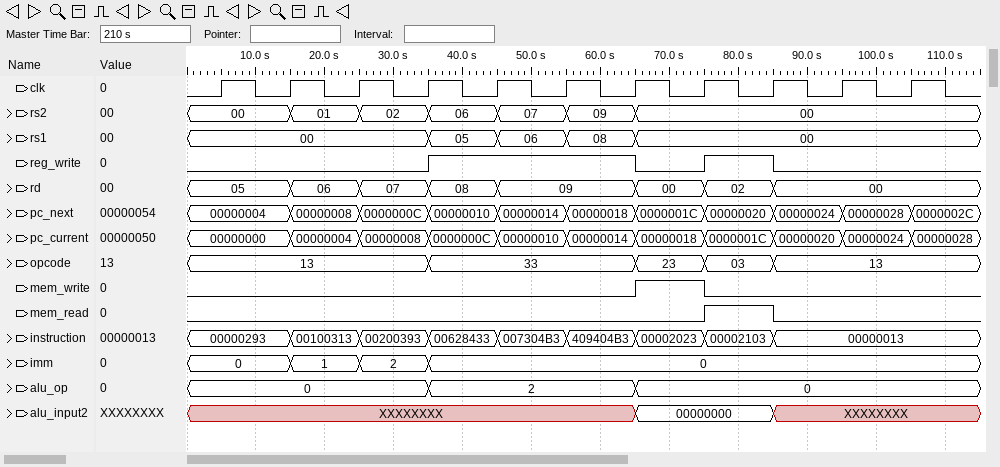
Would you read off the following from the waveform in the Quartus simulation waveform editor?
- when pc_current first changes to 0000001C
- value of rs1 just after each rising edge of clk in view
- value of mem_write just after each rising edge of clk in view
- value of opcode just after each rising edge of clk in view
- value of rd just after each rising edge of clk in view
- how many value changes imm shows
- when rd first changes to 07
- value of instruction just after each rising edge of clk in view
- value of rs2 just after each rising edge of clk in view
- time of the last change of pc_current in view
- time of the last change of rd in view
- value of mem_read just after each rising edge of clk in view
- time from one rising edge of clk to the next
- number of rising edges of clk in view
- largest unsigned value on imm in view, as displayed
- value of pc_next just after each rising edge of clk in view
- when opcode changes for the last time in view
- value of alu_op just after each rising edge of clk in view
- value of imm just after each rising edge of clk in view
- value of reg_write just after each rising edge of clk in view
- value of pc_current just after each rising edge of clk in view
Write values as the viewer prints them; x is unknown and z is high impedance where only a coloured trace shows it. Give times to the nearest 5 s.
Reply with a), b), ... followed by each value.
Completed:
a) 75 s
b) 00, 00, 00, 05, 06, 08, 00, 00, 00, 00, 00
c) 0 0 0 0 0 0 1 0 0 0 0
d) 13, 13, 13, 33, 33, 33, 23, 03, 13, 13, 13
e) 05, 06, 07, 08, 09, 09, 00, 02, 00, 00, 00
f) 3
g) 25 s
h) 00000293, 00100313, 00200393, 00628433, 007304B3, 409404B3, 00002023, 00002103, 00000013, 00000013, 00000013
i) 00, 01, 02, 06, 07, 09, 00, 00, 00, 00, 00
j) 105 s
k) 85 s
l) 0 0 0 0 0 0 0 1 0 0 0
m) 10 s
n) 11
o) 2
p) 00000004, 00000008, 0000000C, 00000010, 00000014, 00000018, 0000001C, 00000020, 00000024, 00000028, 0000002C
q) 85 s
r) 0, 0, 0, 2, 2, 2, 0, 0, 0, 0, 0
s) 0, 1, 2, 0, 0, 0, 0, 0, 0, 0, 0
t) 0 0 0 1 1 1 0 1 0 0 0
u) 00000000, 00000004, 00000008, 0000000C, 00000010, 00000014, 00000018, 0000001C, 00000020, 00000024, 00000028
